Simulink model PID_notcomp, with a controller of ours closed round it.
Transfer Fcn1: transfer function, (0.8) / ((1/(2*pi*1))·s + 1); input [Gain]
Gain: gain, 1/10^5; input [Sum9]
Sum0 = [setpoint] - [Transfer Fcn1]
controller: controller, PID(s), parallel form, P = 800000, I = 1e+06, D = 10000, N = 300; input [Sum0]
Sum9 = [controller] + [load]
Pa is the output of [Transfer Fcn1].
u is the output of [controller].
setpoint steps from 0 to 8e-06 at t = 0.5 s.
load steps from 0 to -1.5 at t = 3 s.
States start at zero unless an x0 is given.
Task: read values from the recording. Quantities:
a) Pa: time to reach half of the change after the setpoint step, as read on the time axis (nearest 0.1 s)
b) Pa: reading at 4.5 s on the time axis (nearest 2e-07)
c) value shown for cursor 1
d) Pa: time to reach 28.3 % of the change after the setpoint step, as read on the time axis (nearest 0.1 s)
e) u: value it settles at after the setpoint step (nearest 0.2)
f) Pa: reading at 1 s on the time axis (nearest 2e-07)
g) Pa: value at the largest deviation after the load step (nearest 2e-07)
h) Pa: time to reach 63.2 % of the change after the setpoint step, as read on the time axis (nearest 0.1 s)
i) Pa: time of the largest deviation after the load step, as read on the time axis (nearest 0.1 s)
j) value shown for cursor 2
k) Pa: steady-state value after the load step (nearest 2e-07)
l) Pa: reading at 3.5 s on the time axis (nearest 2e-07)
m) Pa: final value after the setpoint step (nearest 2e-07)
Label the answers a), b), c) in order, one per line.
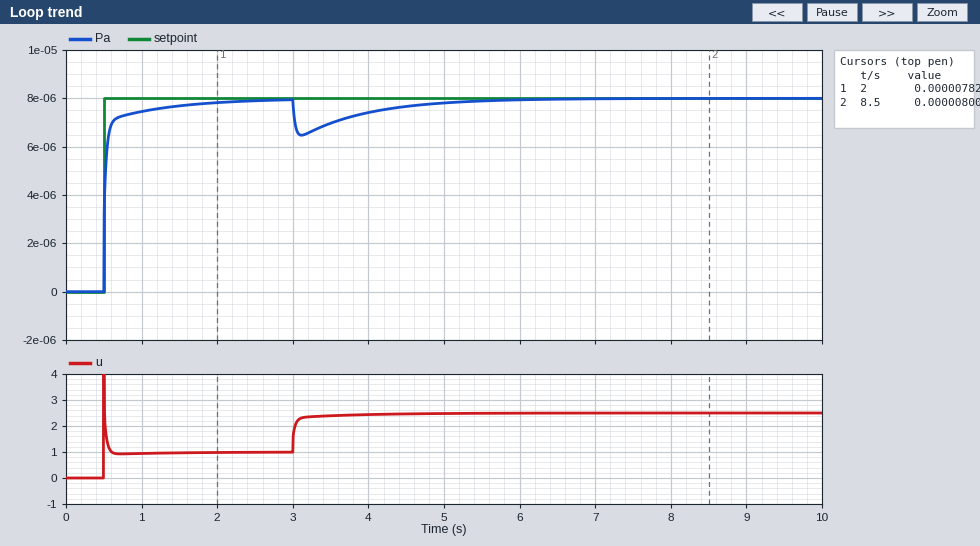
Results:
a) 0.5 s
b) 0.0000076
c) 0.00000782
d) 0.5 s
e) 1.0
f) 0.0000074
g) 0.0000064
h) 0.5 s
i) 3.1 s
j) 0.00000800
k) 0.0000080
l) 0.0000070
m) 0.0000080
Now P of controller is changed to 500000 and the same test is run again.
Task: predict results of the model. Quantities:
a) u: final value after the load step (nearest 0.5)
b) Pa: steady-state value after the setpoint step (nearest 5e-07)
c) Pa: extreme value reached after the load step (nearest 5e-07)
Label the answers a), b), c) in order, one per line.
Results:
a) 2.5
b) 0.0000080
c) 0.0000060
